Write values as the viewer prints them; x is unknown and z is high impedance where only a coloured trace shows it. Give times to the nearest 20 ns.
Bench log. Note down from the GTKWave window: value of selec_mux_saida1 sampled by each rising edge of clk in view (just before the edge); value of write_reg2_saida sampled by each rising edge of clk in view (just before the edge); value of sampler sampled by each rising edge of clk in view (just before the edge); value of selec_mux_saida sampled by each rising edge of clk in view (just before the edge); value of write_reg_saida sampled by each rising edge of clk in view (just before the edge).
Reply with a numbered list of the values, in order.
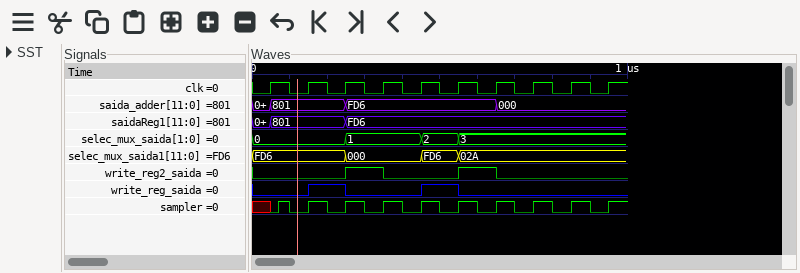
1. FD6, FD6, FD6, 000, 000, FD6, 02A, 02A, 02A, 02A
2. 0 0 0 1 0 0 1 0 0 0
3. x 0 0 0 0 0 0 0 0 0
4. 0, 0, 0, 1, 1, 2, 3, 3, 3, 3
5. 0 0 1 0 0 1 0 0 0 0
